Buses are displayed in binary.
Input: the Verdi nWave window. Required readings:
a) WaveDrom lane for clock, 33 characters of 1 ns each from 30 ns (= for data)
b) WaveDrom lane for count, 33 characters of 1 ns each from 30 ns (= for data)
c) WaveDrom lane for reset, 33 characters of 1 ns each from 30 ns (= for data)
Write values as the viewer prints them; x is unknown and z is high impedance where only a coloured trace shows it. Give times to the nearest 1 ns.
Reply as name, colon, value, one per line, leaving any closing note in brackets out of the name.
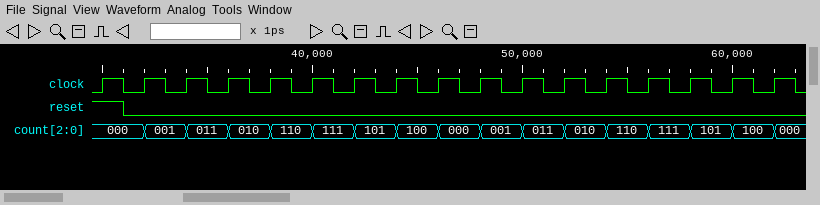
WaveDrom lane for clock, 33 characters of 1 ns each from 30 ns: {name: 'clock', wave: '101010101010101010101010101010101'}
WaveDrom lane for count, 33 characters of 1 ns each from 30 ns: {name: 'count', wave: '=.=.=.=.=.=.=.=.=.=.=.=.=.=.=.=.=', data: '000 001 011 010 110 111 101 100 000 001 011 010 110 111 101 100 000'}
WaveDrom lane for reset, 33 characters of 1 ns each from 30 ns: {name: 'reset', wave: '10...............................'}
